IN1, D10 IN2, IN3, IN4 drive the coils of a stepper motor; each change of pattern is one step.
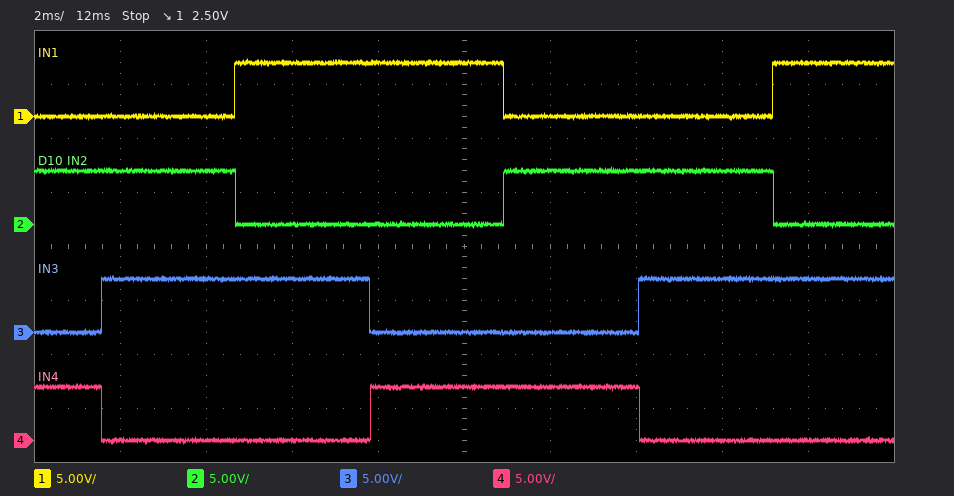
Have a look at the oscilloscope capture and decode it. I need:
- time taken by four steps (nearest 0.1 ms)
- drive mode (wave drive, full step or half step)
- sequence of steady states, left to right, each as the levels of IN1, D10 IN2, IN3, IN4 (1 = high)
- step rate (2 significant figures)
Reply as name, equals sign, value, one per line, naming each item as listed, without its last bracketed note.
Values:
time taken by four steps = 12.5 ms
drive mode = full step
sequence of steady states, left to right, each as the levels of IN1, D10 IN2, IN3, IN4 = 0101 0110 1010 1001 0101 0110 1010
step rate = 320 steps/s
